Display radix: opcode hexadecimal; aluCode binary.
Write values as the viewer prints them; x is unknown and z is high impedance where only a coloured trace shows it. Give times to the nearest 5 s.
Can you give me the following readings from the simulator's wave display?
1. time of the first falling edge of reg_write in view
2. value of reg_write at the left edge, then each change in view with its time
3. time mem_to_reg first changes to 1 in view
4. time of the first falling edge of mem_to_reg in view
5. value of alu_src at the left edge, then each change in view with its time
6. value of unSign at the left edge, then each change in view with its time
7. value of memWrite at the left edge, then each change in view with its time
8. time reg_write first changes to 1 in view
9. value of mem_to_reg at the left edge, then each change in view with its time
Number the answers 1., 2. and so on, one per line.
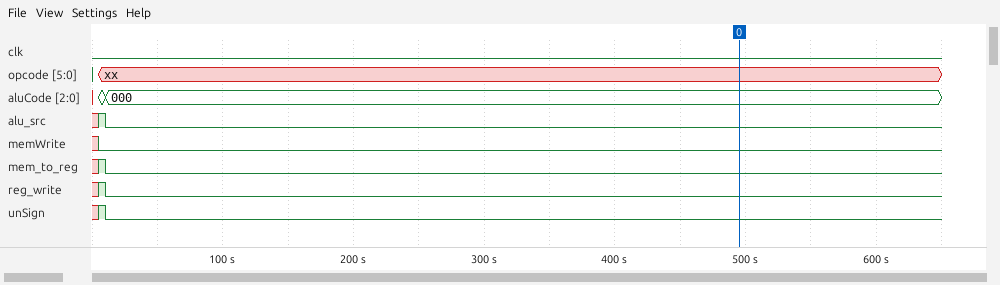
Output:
1. 10 s
2. x, 1 at 5 s, 0 at 10 s
3. 5 s
4. 10 s
5. x, 1 at 5 s, 0 at 10 s
6. x, 1 at 5 s, 0 at 10 s
7. x, 0 at 5 s
8. 5 s
9. x, 1 at 5 s, 0 at 10 s
